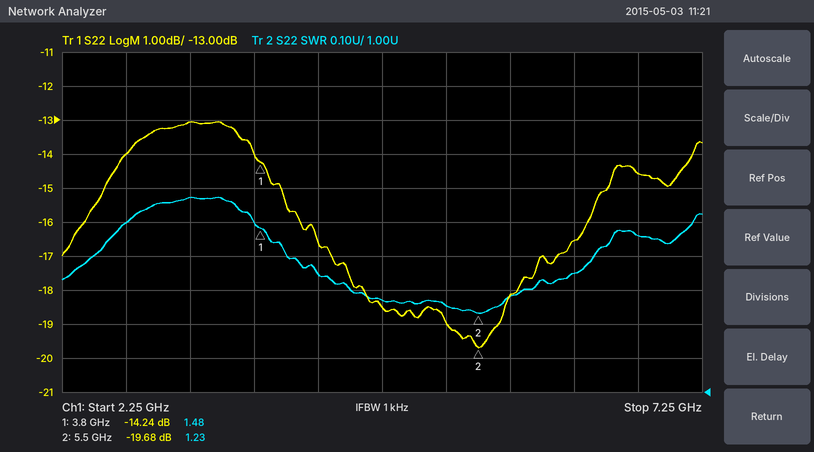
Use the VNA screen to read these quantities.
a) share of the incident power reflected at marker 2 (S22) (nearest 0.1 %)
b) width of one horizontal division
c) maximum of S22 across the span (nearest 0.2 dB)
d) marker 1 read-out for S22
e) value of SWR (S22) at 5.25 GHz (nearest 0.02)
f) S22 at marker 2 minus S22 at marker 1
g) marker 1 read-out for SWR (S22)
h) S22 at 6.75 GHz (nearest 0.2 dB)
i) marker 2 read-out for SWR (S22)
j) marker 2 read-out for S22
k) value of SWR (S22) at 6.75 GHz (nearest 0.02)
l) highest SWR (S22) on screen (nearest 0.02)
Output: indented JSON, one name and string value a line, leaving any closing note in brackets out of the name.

{
  "share of the incident power reflected at marker 2 (S22)": "1.1 %",
  "width of one horizontal division": "500 MHz",
  "maximum of S22 across the span": "-13.0 dB",
  "marker 1 read-out for S22": "-14.24 dB",
  "value of SWR (S22) at 5.25 GHz": "1.26",
  "S22 at marker 2 minus S22 at marker 1": "-5.44 dB",
  "marker 1 read-out for SWR": "1.48",
  "S22 at 6.75 GHz": "-14.6 dB",
  "marker 2 read-out for SWR": "1.23",
  "marker 2 read-out for S22": "-19.68 dB",
  "value of SWR (S22) at 6.75 GHz": "1.46",
  "highest SWR (S22) on screen": "1.58"
}
